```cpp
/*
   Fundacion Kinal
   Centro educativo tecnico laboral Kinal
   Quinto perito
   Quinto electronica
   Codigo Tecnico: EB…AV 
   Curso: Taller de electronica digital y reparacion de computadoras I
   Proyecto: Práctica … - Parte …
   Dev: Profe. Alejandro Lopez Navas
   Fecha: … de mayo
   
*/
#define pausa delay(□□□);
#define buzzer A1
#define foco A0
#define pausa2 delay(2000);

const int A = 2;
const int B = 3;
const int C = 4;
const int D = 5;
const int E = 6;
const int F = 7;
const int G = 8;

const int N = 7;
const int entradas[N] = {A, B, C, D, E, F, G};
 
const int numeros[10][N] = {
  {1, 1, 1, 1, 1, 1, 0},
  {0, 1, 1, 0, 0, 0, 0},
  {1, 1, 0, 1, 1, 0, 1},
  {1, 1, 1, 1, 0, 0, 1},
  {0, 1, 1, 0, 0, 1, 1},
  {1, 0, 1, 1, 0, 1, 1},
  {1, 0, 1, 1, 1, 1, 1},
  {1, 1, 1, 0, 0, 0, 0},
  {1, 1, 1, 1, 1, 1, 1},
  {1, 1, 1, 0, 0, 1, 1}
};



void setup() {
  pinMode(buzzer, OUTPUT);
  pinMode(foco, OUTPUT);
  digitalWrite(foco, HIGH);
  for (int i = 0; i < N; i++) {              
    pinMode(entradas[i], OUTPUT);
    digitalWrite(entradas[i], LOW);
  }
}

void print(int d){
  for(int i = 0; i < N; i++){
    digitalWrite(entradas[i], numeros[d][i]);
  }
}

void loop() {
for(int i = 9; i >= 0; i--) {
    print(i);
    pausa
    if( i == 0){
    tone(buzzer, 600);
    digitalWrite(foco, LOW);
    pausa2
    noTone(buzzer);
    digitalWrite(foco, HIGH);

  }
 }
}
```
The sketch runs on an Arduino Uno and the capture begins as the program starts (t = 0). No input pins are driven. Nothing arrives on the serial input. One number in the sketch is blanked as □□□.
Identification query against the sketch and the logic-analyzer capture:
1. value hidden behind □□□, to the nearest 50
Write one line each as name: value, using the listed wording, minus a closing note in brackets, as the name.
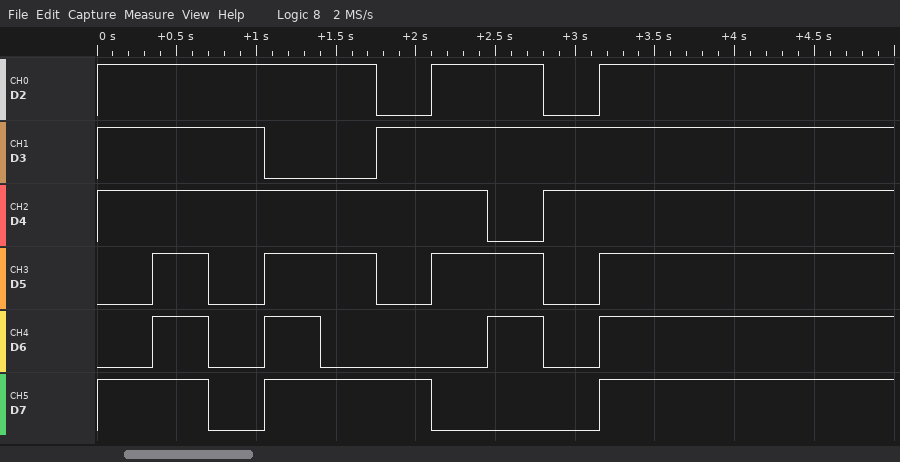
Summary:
value hidden behind □□□, to the nearest 50: 350
